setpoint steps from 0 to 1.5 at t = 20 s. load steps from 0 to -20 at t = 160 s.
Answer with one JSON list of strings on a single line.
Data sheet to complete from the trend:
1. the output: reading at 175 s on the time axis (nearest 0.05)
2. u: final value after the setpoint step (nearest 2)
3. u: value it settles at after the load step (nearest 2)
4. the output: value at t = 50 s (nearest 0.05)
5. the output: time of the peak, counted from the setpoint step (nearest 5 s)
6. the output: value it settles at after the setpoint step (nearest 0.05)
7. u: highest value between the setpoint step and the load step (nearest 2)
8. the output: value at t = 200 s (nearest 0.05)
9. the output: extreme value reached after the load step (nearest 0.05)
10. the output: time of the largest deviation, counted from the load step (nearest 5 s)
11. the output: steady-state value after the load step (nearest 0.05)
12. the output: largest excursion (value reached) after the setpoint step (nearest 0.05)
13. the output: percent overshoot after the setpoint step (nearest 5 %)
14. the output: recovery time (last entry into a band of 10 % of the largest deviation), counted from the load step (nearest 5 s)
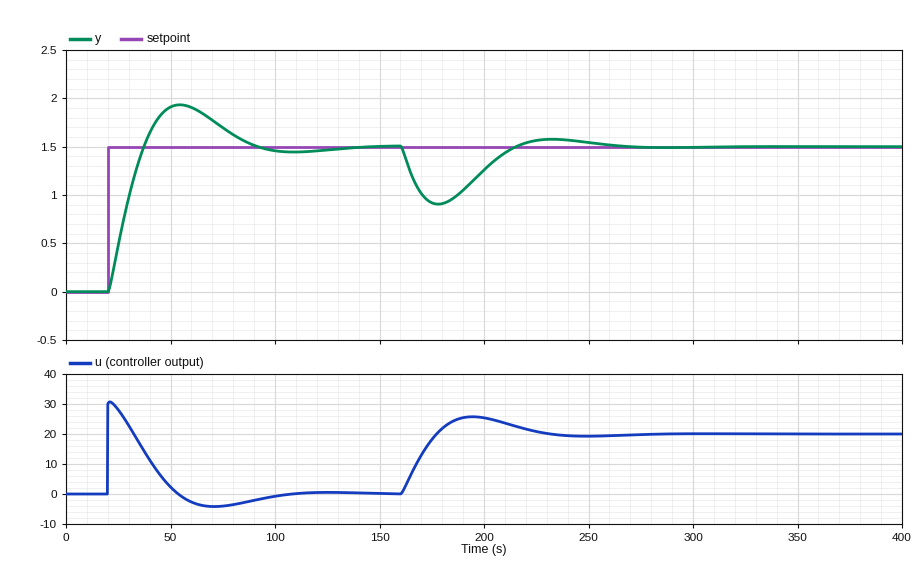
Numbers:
["0.90", "0", "20", "1.90", "35 s", "1.50", "30", "1.25", "0.90", "20 s", "1.50", "1.95", "30 %", "85 s"]
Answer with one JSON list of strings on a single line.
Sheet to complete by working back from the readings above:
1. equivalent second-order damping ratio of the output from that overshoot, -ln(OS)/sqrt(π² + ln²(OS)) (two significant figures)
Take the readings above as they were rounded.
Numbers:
["0.36"]
